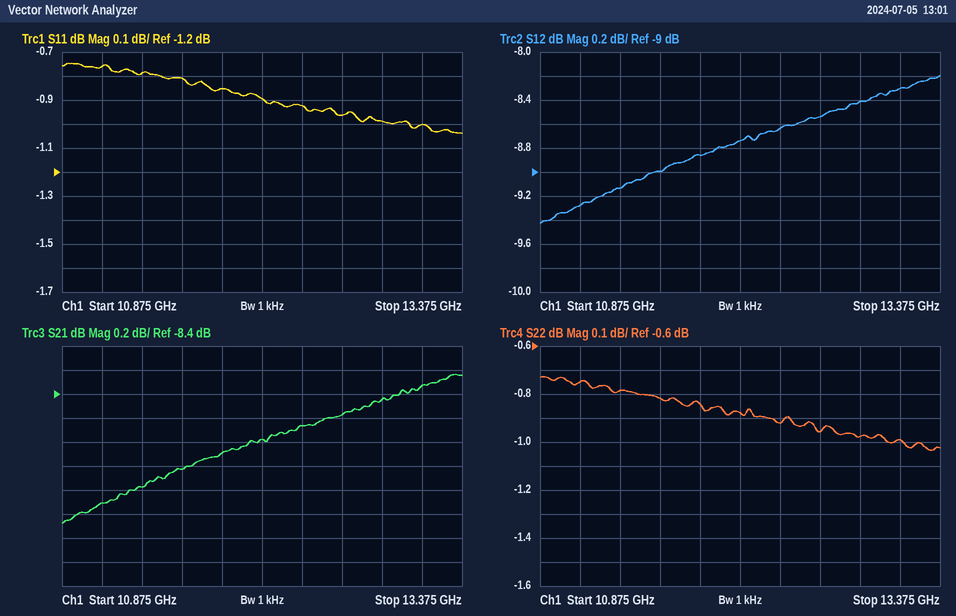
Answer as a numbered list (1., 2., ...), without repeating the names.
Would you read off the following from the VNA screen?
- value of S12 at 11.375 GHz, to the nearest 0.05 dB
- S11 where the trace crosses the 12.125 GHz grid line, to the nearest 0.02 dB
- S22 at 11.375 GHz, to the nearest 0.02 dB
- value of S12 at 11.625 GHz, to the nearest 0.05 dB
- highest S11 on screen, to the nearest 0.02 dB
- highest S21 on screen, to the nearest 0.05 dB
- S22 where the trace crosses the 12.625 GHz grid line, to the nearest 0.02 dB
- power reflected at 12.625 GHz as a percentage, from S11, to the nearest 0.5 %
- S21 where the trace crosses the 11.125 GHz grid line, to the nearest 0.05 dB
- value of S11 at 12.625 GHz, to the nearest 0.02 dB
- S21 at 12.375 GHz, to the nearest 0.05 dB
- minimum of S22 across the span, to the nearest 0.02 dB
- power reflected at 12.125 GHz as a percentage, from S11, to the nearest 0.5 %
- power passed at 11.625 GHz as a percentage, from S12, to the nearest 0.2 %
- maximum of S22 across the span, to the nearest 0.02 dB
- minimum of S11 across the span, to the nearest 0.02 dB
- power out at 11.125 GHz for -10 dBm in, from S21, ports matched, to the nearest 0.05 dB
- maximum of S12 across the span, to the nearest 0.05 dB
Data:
1. -9.15 dB
2. -0.90 dB
3. -0.78 dB
4. -9.00 dB
5. -0.74 dB
6. -8.25 dB
7. -0.96 dB
8. 80.0 %
9. -9.30 dB
10. -0.96 dB
11. -8.65 dB
12. -1.04 dB
13. 81.5 %
14. 12.6 %
15. -0.72 dB
16. -1.04 dB
17. -19.30 dBm
18. -8.20 dB
